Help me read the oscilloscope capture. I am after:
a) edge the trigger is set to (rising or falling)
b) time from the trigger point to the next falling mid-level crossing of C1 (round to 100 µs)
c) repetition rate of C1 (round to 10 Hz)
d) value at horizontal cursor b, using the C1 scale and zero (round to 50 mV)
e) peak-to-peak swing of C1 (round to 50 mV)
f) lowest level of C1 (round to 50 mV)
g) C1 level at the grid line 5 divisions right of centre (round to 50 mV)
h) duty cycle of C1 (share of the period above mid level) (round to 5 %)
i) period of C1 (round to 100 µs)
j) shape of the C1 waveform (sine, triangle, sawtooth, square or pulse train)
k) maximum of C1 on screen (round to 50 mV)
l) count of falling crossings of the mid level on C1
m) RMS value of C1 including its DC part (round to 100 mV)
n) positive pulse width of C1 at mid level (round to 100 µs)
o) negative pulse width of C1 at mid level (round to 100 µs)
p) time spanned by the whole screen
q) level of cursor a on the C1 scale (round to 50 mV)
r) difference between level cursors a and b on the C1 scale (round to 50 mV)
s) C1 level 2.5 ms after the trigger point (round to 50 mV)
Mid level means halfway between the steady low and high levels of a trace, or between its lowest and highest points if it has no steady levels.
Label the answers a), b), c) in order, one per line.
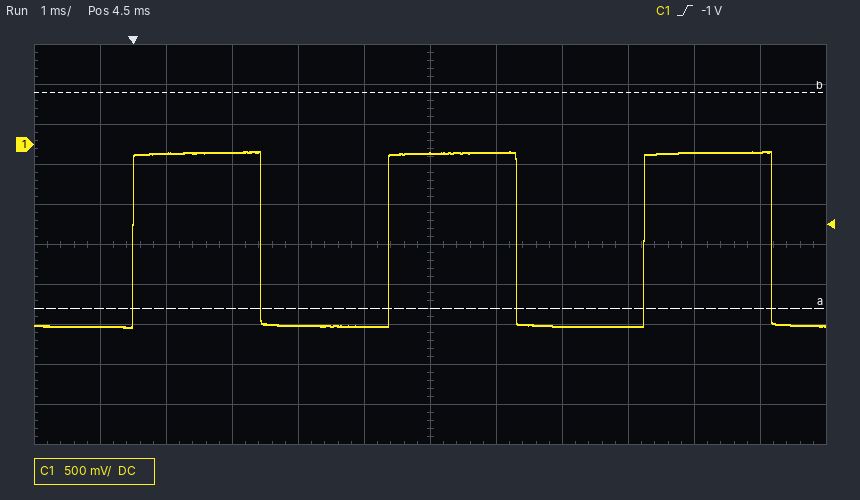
a) rising
b) 1.9 ms
c) 260 Hz
d) 650 mV
e) 2.20 V
f) -2.30 V
g) -100 mV
h) 50 %
i) 3.9 ms
j) square
k) -100 mV
l) 3
m) 1.6 V
n) 1.9 ms
o) 1.9 ms
p) 12 ms
q) -2.05 V
r) 2.70 V
s) -2.25 V
